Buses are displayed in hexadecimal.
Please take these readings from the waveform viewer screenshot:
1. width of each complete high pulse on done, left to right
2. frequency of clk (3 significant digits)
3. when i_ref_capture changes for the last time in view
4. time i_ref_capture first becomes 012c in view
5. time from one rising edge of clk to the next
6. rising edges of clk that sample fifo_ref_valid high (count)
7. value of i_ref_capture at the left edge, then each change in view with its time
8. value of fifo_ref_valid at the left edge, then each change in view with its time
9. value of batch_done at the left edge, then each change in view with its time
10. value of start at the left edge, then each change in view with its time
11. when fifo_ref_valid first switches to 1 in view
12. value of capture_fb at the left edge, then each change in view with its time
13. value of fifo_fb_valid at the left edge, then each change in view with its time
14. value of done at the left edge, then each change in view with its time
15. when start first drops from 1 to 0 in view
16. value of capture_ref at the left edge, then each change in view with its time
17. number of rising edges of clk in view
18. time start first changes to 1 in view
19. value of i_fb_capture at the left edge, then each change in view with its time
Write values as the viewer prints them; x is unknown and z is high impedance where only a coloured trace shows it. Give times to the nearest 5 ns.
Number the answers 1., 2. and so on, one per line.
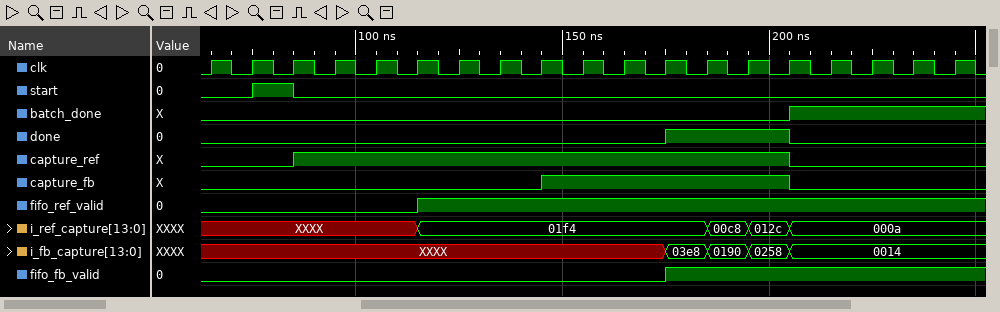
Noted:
1. 30 ns
2. 100 MHz
3. 205 ns
4. 195 ns
5. 10 ns
6. 13
7. XXXX, 01f4 at 115 ns, 00c8 at 185 ns, 012c at 195 ns, 000a at 205 ns
8. 0, 1 at 115 ns
9. 0, 1 at 205 ns
10. 0, 1 at 75 ns, 0 at 85 ns
11. 115 ns
12. 0, 1 at 145 ns, 0 at 205 ns
13. 0, 1 at 175 ns
14. 0, 1 at 175 ns, 0 at 205 ns
15. 85 ns
16. 0, 1 at 85 ns, 0 at 205 ns
17. 19
18. 75 ns
19. XXXX, 03e8 at 175 ns, 0190 at 185 ns, 0258 at 195 ns, 0014 at 205 ns
